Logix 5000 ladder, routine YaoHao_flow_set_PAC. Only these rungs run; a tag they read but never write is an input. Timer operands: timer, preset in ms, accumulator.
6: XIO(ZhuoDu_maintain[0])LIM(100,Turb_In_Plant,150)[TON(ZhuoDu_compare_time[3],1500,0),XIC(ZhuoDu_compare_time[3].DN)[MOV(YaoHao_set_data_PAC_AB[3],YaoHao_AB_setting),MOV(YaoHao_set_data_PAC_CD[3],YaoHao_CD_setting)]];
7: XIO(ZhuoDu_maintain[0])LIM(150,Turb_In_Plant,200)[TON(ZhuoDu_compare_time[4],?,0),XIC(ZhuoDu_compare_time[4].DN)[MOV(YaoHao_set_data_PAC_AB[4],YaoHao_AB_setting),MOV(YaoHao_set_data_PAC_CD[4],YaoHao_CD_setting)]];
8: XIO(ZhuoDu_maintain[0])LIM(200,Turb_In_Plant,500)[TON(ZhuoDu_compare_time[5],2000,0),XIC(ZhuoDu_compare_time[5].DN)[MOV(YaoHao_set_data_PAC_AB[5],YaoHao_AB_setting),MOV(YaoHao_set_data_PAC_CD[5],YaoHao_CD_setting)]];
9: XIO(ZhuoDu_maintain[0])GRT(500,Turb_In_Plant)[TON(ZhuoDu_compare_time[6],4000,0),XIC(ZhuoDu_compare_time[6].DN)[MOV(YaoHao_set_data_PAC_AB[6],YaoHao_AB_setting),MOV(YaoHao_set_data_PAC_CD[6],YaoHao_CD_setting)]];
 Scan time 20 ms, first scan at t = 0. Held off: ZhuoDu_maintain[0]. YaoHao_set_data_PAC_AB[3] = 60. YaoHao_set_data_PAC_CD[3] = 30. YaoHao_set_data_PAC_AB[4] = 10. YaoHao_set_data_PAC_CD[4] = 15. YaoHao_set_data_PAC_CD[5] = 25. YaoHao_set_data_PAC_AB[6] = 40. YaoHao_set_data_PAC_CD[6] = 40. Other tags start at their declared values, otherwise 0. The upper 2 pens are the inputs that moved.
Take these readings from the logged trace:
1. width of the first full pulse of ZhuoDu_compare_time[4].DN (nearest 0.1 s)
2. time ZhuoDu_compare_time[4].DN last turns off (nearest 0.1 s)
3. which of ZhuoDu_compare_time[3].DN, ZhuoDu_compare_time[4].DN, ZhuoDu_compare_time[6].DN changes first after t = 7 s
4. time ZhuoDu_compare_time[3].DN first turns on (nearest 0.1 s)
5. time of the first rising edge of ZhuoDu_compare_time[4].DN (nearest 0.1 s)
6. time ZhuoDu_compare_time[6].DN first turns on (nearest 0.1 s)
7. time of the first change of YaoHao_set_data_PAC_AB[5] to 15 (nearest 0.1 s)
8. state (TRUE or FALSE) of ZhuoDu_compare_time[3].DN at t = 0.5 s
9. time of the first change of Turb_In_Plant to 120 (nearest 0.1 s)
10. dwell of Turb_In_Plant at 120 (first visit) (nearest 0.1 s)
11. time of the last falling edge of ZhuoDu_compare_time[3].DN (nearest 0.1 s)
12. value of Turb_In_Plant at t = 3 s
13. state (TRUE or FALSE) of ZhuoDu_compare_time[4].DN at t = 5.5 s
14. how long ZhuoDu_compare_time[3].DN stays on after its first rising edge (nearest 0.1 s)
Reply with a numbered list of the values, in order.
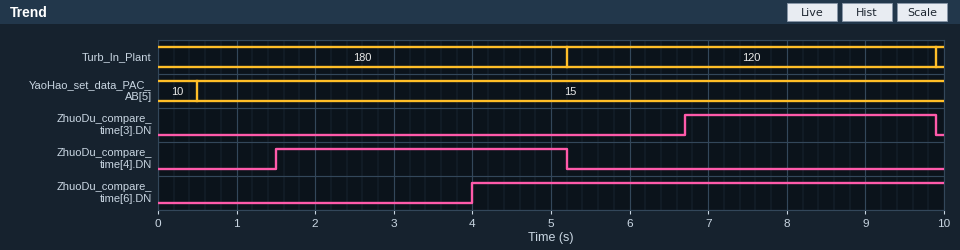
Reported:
1. 3.7 s
2. 5.2 s
3. ZhuoDu_compare_time[3].DN
4. 6.7 s
5. 1.5 s
6. 4.0 s
7. 0.5 s
8. FALSE
9. 5.2 s
10. 4.7 s
11. 9.9 s
12. 180
13. FALSE
14. 3.2 s
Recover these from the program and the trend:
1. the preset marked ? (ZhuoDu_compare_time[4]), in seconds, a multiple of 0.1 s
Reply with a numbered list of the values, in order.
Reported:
1. 1.5 s
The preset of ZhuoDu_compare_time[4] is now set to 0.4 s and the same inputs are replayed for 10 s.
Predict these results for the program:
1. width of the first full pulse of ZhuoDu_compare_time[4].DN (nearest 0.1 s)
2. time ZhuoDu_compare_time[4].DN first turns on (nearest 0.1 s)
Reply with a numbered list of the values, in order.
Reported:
1. 4.8 s
2. 0.4 s
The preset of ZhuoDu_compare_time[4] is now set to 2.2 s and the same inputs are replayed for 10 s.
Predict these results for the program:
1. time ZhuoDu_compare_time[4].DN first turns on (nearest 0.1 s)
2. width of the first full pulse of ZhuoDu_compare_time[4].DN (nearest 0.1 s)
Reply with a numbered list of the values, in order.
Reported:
1. 2.2 s
2. 3.0 s
